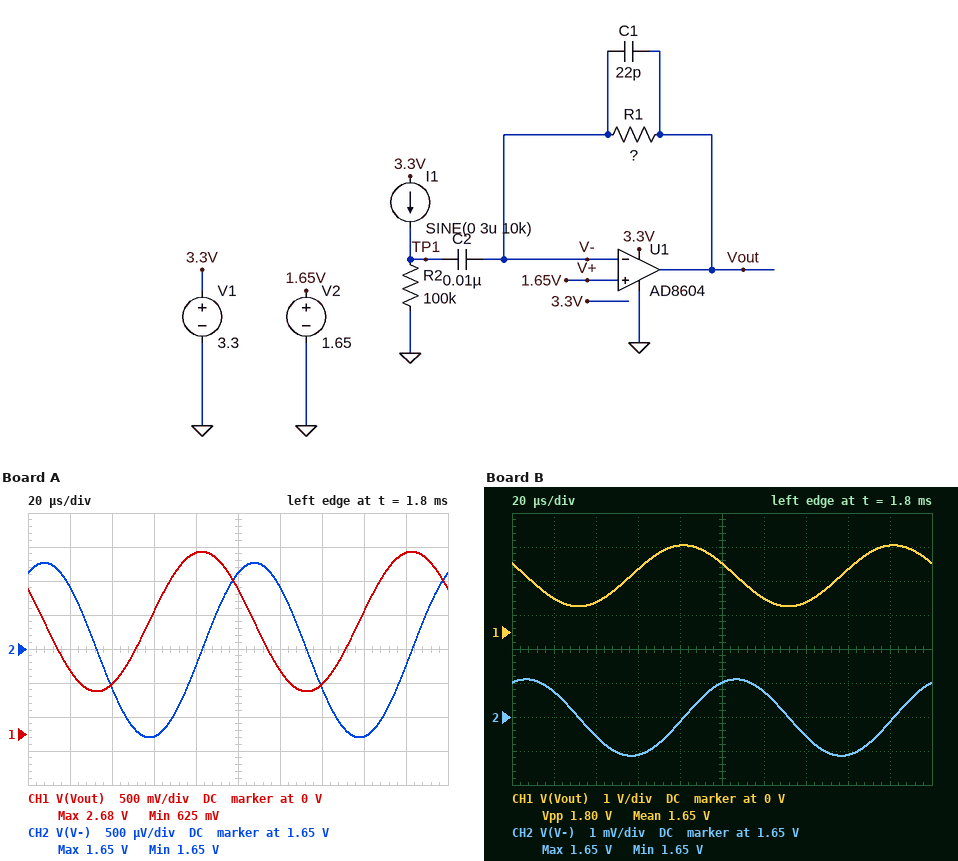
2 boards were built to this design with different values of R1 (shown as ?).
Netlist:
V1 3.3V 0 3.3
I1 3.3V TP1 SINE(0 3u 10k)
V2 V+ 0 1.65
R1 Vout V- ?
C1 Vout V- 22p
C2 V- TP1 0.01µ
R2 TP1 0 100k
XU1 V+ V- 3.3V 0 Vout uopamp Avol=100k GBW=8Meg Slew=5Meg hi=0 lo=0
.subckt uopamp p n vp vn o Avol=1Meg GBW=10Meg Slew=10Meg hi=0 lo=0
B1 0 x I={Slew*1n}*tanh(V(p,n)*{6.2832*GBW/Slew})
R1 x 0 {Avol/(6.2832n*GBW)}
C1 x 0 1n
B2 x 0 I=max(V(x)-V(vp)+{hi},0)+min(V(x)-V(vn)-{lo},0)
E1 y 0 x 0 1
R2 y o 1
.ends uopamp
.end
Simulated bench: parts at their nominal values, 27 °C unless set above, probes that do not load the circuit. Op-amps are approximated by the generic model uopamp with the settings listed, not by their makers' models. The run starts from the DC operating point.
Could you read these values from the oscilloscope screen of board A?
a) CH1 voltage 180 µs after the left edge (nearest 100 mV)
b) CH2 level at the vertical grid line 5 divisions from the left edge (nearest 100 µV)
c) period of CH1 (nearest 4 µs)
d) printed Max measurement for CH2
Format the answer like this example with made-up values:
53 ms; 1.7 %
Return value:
2.7 V; 1.6511 V; 100 µs; 1.65 V
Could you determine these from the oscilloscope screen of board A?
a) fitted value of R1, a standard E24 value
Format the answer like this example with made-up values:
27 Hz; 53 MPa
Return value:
390 kΩ
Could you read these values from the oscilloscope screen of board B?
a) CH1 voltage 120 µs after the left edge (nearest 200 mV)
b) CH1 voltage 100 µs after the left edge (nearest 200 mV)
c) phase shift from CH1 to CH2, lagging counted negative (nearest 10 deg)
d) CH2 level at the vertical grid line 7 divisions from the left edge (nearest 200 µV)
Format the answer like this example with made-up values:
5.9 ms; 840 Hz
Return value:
1.0 V; 2.0 V; -90 deg; 1.6494 V
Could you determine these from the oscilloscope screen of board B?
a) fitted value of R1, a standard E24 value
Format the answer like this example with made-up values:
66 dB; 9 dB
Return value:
330 kΩ
